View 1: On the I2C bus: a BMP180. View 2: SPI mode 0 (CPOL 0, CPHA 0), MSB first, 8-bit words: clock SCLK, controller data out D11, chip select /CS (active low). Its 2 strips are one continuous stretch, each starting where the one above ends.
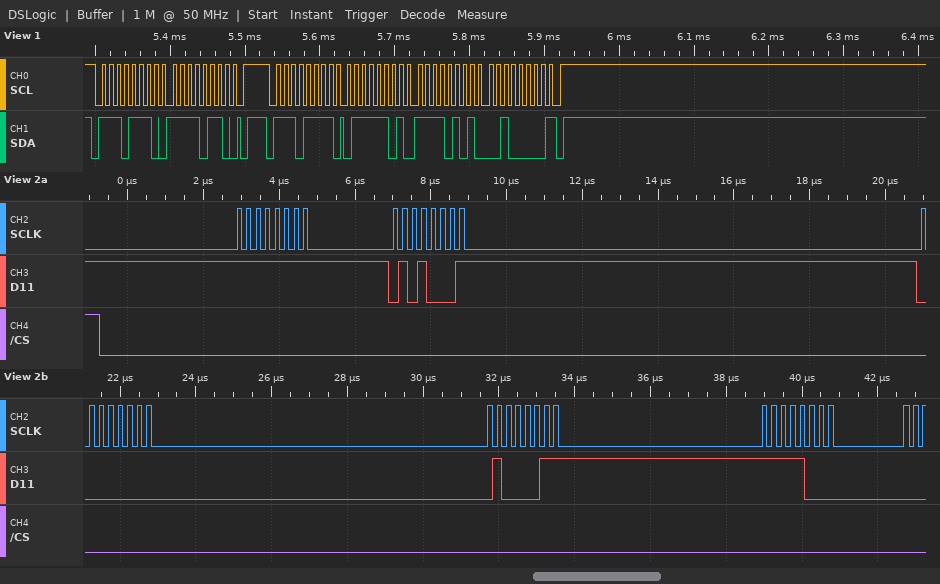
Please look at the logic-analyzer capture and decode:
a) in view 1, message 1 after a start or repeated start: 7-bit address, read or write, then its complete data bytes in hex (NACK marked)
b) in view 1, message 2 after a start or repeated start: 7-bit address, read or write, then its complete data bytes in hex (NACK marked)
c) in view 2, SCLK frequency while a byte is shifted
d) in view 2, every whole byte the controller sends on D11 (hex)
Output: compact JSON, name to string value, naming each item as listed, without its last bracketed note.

{"in view 1, message 1 after a start or repeated start: 7-bit address, read or write, then its complete data bytes in hex": "0x77 write: F6", "in view 1, message 2 after a start or repeated start: 7-bit address, read or write, then its complete data bytes in hex": "0x77 read: 7D F5 20 NACK", "in view 2, SCLK frequency while a byte is shifted": "4 MHz", "in view 2, every whole byte the controller sends on D11": "FF 51 00 43 F8"}
